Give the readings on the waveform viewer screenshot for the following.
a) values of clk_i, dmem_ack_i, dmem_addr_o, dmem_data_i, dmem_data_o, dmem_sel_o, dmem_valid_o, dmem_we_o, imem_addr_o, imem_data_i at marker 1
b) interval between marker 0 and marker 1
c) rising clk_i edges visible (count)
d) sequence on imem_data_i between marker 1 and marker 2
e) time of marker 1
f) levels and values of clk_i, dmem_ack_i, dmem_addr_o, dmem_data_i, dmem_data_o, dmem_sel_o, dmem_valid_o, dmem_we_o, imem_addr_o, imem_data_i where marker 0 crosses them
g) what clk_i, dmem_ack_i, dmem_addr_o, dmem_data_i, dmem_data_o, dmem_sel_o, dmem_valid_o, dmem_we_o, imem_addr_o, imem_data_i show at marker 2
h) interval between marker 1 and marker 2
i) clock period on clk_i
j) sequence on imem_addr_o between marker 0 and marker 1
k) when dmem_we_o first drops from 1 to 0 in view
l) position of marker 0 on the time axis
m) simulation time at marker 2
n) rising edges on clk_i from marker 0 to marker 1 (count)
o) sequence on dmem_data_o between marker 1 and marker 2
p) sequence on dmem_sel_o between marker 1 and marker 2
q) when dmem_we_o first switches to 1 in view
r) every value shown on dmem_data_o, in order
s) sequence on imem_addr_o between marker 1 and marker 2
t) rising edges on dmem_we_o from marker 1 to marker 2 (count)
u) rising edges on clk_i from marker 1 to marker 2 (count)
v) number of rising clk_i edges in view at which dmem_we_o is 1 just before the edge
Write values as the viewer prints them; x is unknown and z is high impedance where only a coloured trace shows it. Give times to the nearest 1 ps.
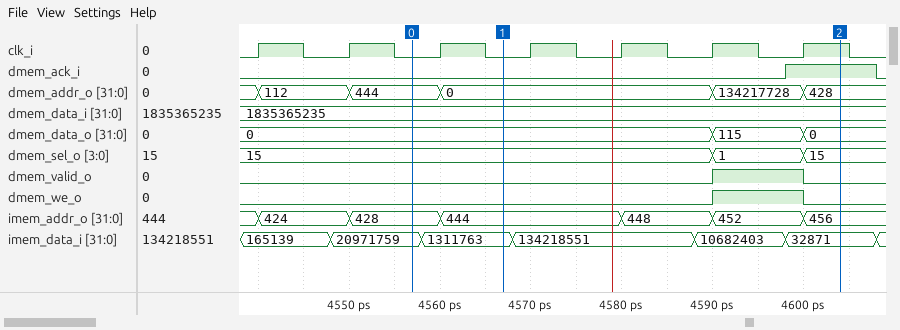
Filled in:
clk_i=0, dmem_ack_i=0, dmem_addr_o=0, dmem_data_i=1835365235, dmem_data_o=0, dmem_sel_o=15, dmem_valid_o=0, dmem_we_o=0, imem_addr_o=444, imem_data_i=1311763
10 ps
7
1311763, 134218551, 10682403, 32871
4567 ps
clk_i=0, dmem_ack_i=0, dmem_addr_o=444, dmem_data_i=1835365235, dmem_data_o=0, dmem_sel_o=15, dmem_valid_o=0, dmem_we_o=0, imem_addr_o=428, imem_data_i=20971759
clk_i=1, dmem_ack_i=1, dmem_addr_o=428, dmem_data_i=1835365235, dmem_data_o=0, dmem_sel_o=15, dmem_valid_o=0, dmem_we_o=0, imem_addr_o=456, imem_data_i=32871
37 ps
10 ps
428, 444
4600 ps
4557 ps
4604 ps
1
0, 115, 0
15, 1, 15
4590 ps
0, 115, 0
444, 448, 452, 456
1
4
1
